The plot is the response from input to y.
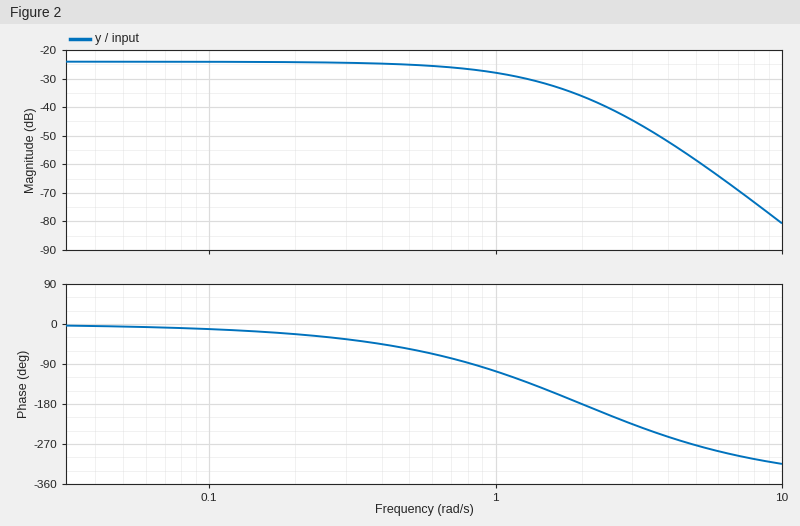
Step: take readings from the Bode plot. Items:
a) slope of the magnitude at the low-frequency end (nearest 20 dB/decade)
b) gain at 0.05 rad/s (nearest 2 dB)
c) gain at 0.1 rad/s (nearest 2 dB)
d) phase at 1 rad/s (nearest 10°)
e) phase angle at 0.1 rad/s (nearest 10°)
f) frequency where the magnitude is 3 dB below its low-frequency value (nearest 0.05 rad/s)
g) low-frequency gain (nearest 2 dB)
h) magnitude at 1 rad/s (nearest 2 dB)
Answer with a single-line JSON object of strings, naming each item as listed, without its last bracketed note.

{"slope of the magnitude at the low-frequency end": "0 dB/decade", "gain at 0.05 rad/s": "-24 dB", "gain at 0.1 rad/s": "-24 dB", "phase at 1 rad/s": "-110°", "phase angle at 0.1 rad/s": "-10°", "frequency where the magnitude is 3 dB below its low-frequency value": "0.85 rad/s", "low-frequency gain": "-24 dB", "magnitude at 1 rad/s": "-28 dB"}
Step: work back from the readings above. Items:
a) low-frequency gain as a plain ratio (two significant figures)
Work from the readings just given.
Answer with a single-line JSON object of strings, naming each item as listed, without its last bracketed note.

{"low-frequency gain as a plain ratio": "0.063"}
